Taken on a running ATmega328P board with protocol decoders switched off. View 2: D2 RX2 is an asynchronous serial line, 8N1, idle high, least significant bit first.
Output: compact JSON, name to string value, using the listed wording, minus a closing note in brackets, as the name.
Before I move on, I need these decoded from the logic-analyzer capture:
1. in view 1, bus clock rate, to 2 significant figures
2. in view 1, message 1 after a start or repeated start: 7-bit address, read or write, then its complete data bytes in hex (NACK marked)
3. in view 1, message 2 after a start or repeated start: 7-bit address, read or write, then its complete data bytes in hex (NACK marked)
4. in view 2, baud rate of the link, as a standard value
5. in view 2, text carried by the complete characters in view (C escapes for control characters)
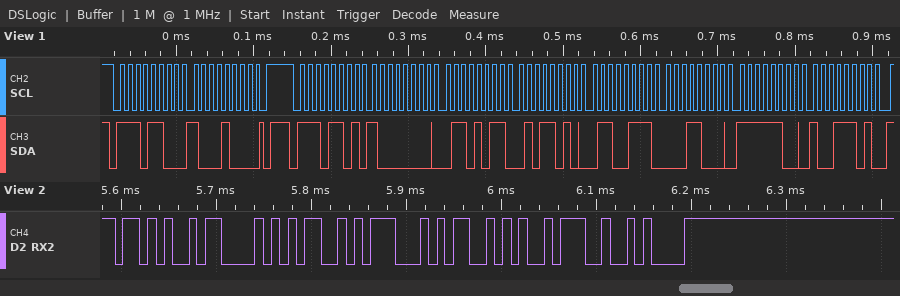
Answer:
{"in view 1, bus clock rate, to 2 significant figures": "100 kHz", "in view 1, message 1 after a start or repeated start: 7-bit address, read or write, then its complete data bytes in hex": "0x76 write: 88", "in view 1, message 2 after a start or repeated start: 7-bit address, read or write, then its complete data bytes in hex": "0x76 read: 80 6B 5A 67 18 FC 9D", "in view 2, baud rate of the link, as a standard value": "115200 baud", "in view 2, text carried by the complete characters in view": "\"+CMGS:\\n\""}
